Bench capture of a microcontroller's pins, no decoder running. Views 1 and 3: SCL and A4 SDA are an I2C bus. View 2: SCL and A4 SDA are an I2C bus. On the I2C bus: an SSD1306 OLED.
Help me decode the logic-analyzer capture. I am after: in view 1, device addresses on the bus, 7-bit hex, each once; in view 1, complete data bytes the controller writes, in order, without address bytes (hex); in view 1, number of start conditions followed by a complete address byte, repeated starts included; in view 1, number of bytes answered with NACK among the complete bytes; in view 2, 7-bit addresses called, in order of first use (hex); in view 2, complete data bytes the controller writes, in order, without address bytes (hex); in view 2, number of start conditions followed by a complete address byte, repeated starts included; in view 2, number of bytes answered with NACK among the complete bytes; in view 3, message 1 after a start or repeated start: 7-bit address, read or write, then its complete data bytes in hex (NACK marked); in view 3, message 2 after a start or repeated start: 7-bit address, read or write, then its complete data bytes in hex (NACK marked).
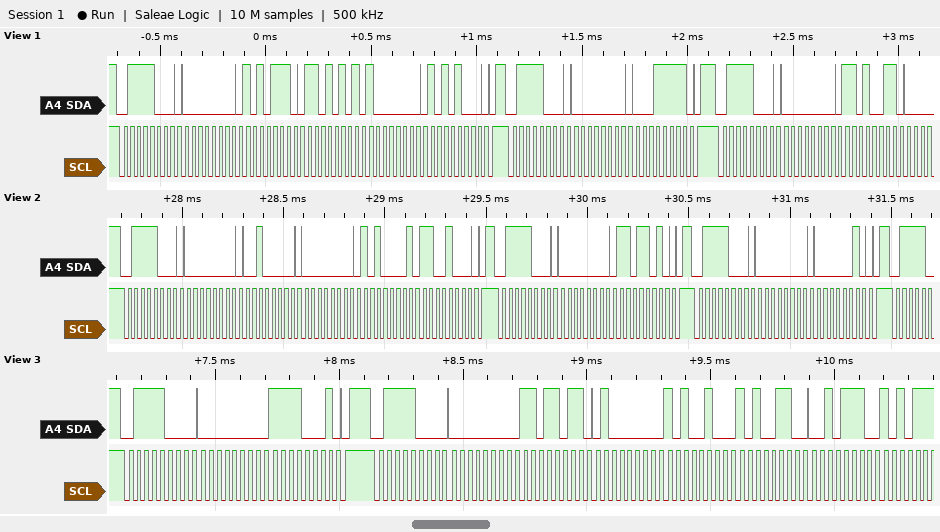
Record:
0x3C
00 AE D5 80 A8 00 1F 00 D3
3
0
0x3C
00 20 00 A1 C8 00 DA 00 02
3
0
0x3C write: 00 F1
0x3C write: 00 DB 40 A4 A6 2E
